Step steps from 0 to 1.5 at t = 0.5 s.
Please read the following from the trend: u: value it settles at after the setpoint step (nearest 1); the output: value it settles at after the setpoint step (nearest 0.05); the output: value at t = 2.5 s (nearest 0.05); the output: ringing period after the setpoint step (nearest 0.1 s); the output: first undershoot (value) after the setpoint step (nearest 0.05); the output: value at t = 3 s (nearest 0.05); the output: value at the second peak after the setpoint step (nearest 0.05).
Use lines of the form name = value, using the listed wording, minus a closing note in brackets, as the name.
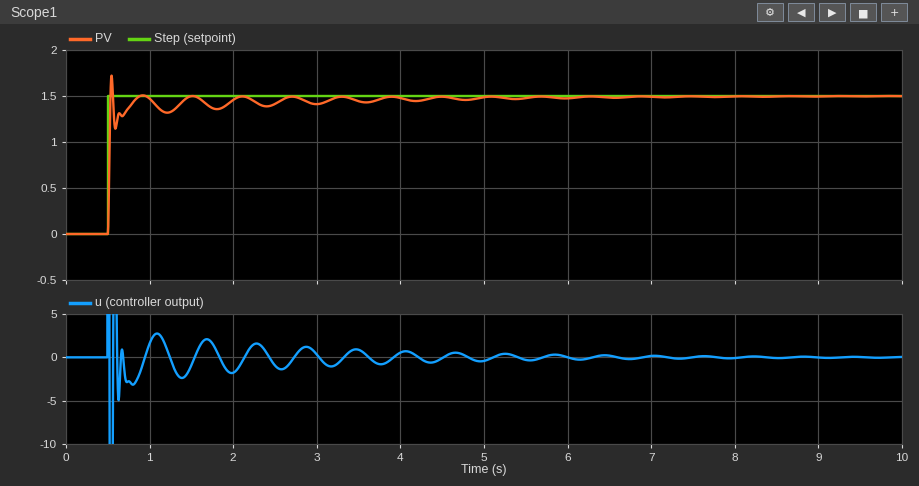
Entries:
u: value it settles at after the setpoint step = 0
the output: value it settles at after the setpoint step = 1.50
the output: value at t = 2.5 s = 1.40
the output: ringing period after the setpoint step = 0.4 s
the output: first undershoot (value) after the setpoint step = 1.15
the output: value at t = 3 s = 1.40
the output: value at the second peak after the setpoint step = 1.50
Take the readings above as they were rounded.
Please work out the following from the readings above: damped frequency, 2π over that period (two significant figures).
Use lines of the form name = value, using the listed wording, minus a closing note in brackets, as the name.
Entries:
damped frequency, 2π over that period = 16 rad/s
